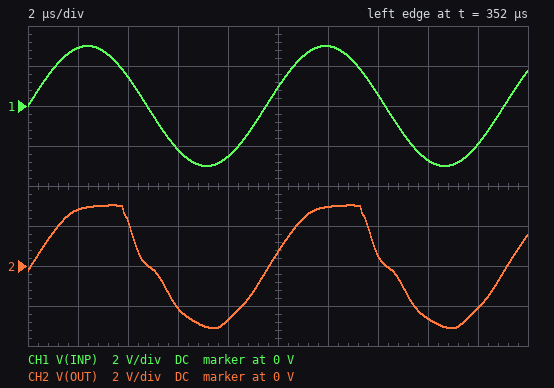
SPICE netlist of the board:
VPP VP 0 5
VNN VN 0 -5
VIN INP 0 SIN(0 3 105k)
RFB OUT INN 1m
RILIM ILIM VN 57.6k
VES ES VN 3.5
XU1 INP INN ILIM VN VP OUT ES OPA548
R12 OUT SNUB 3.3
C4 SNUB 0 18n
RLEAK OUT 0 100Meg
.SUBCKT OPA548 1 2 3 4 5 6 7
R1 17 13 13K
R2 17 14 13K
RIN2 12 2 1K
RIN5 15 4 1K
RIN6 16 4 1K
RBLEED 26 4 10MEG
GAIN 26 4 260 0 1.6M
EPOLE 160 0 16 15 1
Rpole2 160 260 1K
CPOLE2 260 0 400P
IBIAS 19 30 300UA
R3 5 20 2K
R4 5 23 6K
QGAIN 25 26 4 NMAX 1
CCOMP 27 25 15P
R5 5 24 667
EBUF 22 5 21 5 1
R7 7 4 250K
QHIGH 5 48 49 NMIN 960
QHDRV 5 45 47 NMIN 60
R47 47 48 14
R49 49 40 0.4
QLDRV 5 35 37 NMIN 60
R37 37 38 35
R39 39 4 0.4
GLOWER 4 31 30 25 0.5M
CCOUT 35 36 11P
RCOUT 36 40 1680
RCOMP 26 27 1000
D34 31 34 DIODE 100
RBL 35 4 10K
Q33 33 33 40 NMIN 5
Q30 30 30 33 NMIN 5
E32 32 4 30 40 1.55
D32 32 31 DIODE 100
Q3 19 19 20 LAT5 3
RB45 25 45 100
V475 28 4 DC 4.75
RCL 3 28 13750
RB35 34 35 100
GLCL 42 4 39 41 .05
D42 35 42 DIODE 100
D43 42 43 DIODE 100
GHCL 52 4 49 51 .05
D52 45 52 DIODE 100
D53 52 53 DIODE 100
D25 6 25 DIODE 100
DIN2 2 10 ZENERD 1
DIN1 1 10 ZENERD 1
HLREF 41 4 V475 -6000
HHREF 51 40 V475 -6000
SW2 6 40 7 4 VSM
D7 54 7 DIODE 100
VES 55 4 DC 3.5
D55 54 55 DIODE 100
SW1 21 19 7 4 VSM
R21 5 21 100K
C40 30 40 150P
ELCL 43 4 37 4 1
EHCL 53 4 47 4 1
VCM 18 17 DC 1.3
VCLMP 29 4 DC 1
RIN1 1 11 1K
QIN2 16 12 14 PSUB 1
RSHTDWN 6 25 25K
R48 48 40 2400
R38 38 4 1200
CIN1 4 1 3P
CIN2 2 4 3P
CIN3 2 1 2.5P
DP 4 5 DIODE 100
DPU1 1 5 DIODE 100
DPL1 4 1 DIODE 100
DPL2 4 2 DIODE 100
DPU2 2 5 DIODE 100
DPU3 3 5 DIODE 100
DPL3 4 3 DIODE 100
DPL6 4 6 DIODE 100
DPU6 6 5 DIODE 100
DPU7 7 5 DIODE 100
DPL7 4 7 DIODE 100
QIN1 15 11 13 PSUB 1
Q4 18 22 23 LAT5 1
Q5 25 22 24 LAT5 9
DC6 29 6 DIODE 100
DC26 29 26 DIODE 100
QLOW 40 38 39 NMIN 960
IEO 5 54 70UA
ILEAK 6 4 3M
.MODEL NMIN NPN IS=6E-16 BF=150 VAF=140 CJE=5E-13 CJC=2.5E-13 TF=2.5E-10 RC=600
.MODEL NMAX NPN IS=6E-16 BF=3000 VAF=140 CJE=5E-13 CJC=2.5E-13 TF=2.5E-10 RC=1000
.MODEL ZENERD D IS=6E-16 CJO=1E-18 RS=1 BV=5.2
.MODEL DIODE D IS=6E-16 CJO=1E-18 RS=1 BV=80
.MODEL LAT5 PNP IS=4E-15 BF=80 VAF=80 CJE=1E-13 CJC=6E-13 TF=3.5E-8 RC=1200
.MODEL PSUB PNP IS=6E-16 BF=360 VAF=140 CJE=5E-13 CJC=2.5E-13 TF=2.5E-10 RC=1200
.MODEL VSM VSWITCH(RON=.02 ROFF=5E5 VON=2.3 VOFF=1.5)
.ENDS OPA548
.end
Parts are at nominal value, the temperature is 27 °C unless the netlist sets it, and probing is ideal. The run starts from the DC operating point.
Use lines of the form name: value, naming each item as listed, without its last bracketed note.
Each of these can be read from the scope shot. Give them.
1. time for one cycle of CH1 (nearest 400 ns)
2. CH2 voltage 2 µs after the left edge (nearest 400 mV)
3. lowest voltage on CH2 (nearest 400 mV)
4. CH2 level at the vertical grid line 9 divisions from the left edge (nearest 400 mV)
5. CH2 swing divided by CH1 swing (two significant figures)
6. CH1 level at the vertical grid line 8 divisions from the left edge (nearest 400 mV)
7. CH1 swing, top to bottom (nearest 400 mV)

time for one cycle of CH1: 9.6 µs
CH2 voltage 2 µs after the left edge: 2.8 V
lowest voltage on CH2: -3.2 V
CH2 level at the vertical grid line 9 divisions from the left edge: -2.0 V
CH2 swing divided by CH1 swing: 1.0
CH1 level at the vertical grid line 8 divisions from the left edge: -2.8 V
CH1 swing, top to bottom: 6.0 V
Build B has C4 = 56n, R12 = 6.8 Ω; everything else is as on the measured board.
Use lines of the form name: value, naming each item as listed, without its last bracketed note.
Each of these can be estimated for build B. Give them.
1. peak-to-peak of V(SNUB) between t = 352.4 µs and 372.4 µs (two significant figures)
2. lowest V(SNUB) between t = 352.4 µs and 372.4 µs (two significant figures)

peak-to-peak of V(SNUB) between t = 352.4 µs and 372.4 µs: 6.0 V
lowest V(SNUB) between t = 352.4 µs and 372.4 µs: -3.0 V
